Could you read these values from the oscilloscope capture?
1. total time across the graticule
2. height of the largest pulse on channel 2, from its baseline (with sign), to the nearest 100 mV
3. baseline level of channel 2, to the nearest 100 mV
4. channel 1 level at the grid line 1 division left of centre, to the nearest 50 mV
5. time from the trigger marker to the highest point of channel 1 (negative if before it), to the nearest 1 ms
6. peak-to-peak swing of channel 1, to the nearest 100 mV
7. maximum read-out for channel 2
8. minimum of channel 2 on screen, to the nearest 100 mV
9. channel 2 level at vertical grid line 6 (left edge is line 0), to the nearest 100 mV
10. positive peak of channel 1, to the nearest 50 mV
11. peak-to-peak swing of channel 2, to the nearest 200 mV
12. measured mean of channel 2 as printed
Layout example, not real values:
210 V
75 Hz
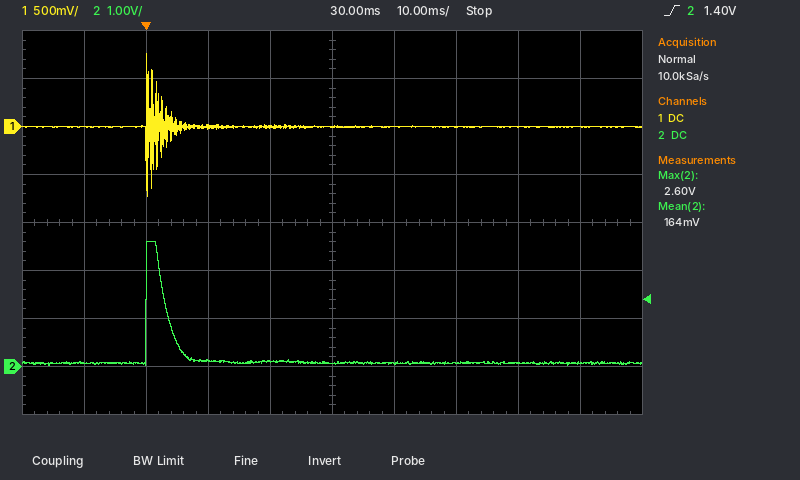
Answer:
100 ms
+2.5 V
100 mV
0 mV
0 ms
1.50 V
2.60 V
0.0 V
100 mV
750 mV
2.6 V
164 mV
